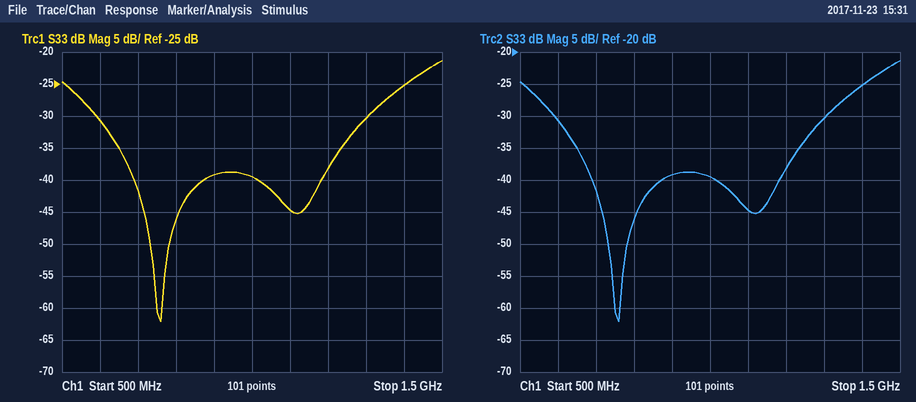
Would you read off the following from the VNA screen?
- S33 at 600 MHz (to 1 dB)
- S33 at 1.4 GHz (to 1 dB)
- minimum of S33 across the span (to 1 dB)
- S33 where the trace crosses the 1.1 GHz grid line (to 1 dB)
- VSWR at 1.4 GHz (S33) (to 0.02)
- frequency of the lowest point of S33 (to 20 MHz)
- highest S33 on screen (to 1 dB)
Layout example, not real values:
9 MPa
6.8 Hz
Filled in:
-31 dB
-25 dB
-62 dB
-45 dB
1.12
760 MHz
-21 dB
